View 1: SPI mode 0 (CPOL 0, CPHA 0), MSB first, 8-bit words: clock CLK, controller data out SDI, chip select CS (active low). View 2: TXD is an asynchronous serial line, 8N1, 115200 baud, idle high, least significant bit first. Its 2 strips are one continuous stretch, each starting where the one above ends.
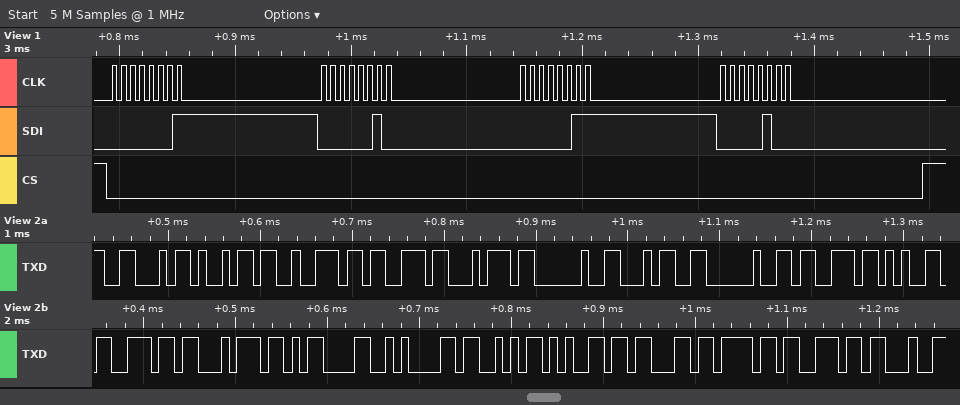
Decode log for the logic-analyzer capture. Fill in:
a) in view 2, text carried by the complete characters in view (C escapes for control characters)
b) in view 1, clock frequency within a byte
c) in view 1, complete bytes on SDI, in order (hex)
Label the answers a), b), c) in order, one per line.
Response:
a) "First 4 sent\r\nSecon"
b) 125 kHz
c) 0x01 0x02 0x03 0x04
